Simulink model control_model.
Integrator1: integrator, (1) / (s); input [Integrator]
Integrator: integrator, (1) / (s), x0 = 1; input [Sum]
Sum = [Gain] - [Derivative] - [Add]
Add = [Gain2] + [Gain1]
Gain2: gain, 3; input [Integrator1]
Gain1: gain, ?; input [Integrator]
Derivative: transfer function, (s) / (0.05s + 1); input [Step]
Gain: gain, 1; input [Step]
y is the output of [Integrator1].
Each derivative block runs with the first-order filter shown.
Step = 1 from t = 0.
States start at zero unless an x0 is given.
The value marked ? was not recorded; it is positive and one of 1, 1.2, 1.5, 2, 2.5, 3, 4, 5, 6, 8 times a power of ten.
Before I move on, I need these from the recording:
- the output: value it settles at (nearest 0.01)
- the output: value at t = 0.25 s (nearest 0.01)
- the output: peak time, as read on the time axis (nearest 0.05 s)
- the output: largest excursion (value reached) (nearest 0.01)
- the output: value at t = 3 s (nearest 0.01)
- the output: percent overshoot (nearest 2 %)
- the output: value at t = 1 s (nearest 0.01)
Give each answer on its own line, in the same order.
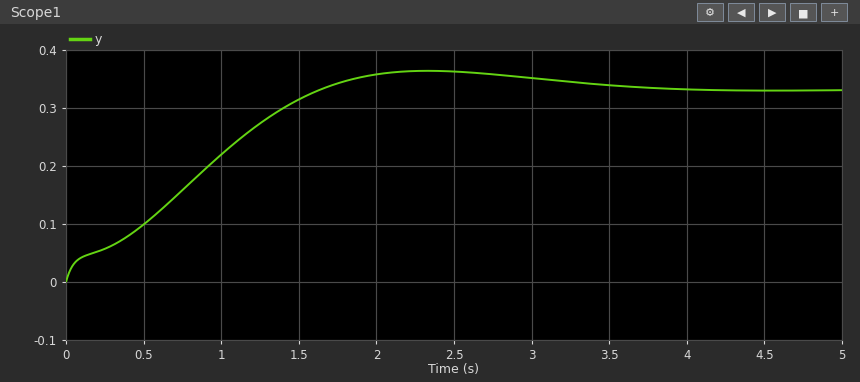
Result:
0.33
0.06
2.35 s
0.36
0.35
10 %
0.22
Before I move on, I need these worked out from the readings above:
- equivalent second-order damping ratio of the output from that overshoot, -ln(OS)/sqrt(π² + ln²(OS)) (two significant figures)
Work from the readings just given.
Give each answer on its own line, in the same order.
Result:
0.59
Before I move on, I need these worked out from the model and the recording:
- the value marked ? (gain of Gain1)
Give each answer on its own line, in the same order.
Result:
2
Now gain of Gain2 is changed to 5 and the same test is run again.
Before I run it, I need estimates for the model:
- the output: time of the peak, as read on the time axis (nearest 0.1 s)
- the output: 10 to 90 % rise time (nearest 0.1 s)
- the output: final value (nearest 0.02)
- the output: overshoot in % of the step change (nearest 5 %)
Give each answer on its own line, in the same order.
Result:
1.7 s
1.0 s
0.20
15 %
